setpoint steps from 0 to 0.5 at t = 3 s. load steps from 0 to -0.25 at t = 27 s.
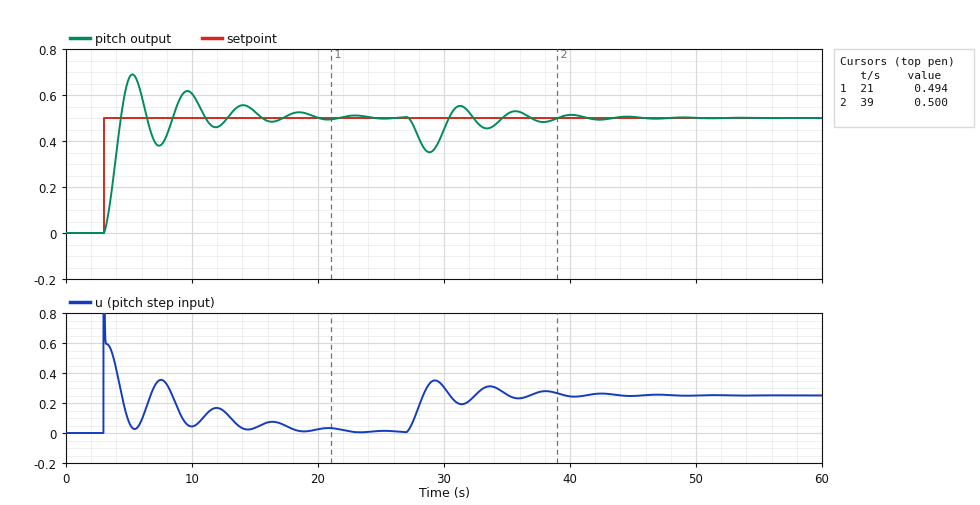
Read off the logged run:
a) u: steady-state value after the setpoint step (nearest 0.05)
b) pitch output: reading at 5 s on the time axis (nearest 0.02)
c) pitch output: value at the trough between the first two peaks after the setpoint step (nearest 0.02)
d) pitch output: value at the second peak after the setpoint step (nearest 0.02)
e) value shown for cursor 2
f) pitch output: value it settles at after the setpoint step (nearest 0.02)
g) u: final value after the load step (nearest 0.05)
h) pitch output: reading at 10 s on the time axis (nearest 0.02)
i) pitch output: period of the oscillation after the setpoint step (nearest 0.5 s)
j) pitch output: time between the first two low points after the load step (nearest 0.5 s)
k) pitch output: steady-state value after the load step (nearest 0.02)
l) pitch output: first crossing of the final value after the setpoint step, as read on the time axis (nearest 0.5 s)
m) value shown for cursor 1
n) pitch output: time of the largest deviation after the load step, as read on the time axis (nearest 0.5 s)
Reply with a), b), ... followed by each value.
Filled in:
a) 0.00
b) 0.68
c) 0.38
d) 0.62
e) 0.500
f) 0.50
g) 0.25
h) 0.60
i) 4.5 s
j) 4.5 s
k) 0.50
l) 4.5 s
m) 0.494
n) 29.0 s
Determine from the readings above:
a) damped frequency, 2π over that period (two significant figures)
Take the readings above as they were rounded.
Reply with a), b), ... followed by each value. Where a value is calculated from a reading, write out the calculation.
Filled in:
a) 2π / 4.5 = 1.4 rad/s
